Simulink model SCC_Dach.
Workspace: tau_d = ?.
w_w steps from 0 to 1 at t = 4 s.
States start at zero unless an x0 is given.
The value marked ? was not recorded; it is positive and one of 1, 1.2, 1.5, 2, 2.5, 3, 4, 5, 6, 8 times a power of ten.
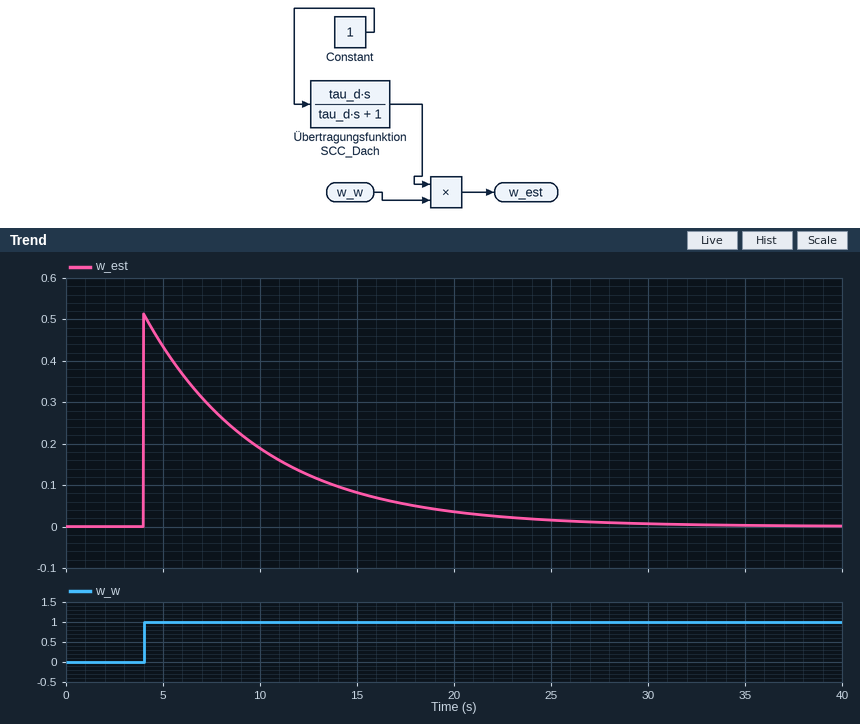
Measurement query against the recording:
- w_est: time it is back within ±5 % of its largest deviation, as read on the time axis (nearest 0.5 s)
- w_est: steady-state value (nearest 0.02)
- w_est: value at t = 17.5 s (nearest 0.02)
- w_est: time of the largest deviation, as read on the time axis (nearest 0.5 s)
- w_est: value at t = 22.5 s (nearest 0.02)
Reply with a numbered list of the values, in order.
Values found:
1. 22.0 s
2. 0.00
3. 0.06
4. 4.0 s
5. 0.02
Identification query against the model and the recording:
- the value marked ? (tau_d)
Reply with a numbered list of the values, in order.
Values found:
1. 6
